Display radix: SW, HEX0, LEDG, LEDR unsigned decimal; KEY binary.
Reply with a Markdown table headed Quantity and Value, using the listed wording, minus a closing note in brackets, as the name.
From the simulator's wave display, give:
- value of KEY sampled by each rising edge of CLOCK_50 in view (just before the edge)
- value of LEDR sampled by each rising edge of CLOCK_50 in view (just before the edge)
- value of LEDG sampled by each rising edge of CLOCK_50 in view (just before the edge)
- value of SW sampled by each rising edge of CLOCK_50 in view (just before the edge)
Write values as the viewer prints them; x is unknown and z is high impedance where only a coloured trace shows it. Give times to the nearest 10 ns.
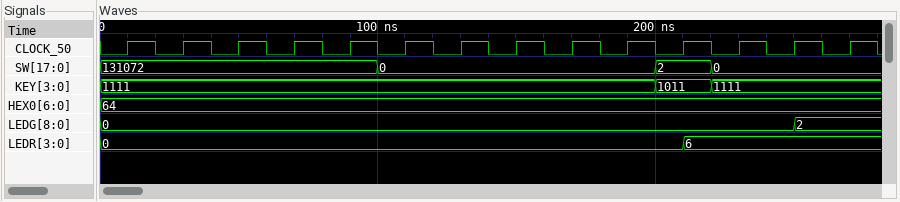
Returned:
| Quantity | Value |
|---|---|
| value of KEY sampled by each rising edge of CLOCK_50 in view | 1111, 1111, 1111, 1111, 1111, 1111, 1111, 1111, 1111, 1111, 1011, 1111, 1111, 1111 |
| value of LEDR sampled by each rising edge of CLOCK_50 in view | 0, 0, 0, 0, 0, 0, 0, 0, 0, 0, 0, 6, 6, 6 |
| value of LEDG sampled by each rising edge of CLOCK_50 in view | 0, 0, 0, 0, 0, 0, 0, 0, 0, 0, 0, 0, 0, 2 |
| value of SW sampled by each rising edge of CLOCK_50 in view | 131072, 131072, 131072, 131072, 131072, 0, 0, 0, 0, 0, 2, 0, 0, 0 |
